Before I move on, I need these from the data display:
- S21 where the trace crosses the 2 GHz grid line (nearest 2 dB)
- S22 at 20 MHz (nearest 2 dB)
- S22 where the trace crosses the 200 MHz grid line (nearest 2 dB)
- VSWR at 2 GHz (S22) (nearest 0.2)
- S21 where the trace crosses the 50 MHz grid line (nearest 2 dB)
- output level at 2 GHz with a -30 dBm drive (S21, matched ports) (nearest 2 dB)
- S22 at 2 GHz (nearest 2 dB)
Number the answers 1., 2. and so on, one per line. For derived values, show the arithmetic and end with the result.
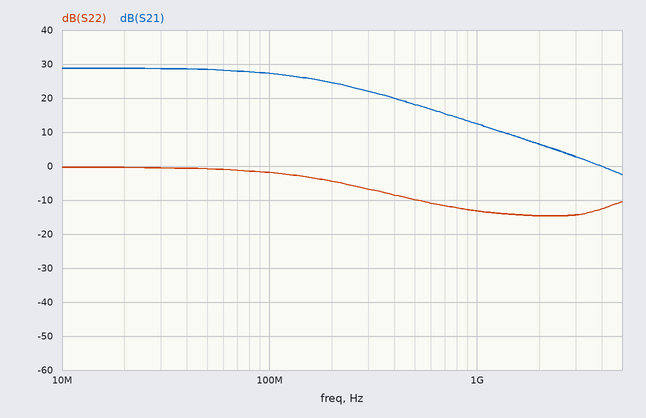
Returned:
1. 6 dB
2. 0 dB
3. -4 dB
4. |Γ| = 10^(-14/20) = 0.1995; VSWR = (1 + 0.1995)/(1 − 0.1995) ≈ 1.50, so 1.4 to the nearest 0.2
5. 28 dB
6. -30 dBm + (6 dB) = -24 dBm
7. -14 dB
